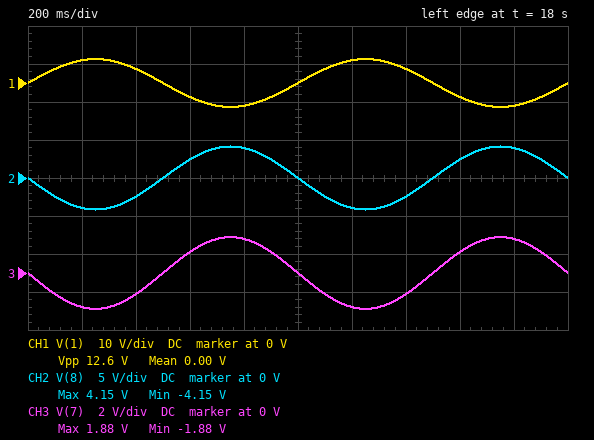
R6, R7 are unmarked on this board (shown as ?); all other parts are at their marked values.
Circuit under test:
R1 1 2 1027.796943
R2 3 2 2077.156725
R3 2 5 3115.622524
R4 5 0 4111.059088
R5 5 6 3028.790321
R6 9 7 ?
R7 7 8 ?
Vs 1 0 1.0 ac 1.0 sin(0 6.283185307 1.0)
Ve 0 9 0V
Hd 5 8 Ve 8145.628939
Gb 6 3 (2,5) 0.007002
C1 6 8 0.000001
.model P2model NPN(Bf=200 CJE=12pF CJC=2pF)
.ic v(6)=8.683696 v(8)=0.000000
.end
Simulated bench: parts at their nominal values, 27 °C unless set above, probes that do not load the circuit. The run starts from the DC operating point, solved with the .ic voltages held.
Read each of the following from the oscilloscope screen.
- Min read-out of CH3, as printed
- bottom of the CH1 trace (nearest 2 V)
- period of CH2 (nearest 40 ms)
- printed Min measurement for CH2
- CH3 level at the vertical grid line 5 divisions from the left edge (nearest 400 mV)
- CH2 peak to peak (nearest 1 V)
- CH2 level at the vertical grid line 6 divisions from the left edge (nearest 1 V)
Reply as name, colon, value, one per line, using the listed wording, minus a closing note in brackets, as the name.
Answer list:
Min read-out of CH3, as printed: -1.88 V
bottom of the CH1 trace: -6 V
period of CH2: 1.00 s
printed Min measurement for CH2: -4.15 V
CH3 level at the vertical grid line 5 divisions from the left edge: 0 V
CH2 peak to peak: 8 V
CH2 level at the vertical grid line 6 divisions from the left edge: -4 V
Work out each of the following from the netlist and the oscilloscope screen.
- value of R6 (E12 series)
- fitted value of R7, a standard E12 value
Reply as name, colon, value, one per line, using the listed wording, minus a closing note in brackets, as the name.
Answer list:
value of R6: 1.5 kΩ
fitted value of R7, a standard E12 value: 1.8 kΩ
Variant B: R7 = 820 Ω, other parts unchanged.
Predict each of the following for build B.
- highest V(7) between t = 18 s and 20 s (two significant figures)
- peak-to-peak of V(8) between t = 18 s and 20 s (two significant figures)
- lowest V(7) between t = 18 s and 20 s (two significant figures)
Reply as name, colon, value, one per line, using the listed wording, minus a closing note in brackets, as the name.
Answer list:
highest V(7) between t = 18 s and 20 s: 1.5 V
peak-to-peak of V(8) between t = 18 s and 20 s: 4.7 V
lowest V(7) between t = 18 s and 20 s: -1.5 V
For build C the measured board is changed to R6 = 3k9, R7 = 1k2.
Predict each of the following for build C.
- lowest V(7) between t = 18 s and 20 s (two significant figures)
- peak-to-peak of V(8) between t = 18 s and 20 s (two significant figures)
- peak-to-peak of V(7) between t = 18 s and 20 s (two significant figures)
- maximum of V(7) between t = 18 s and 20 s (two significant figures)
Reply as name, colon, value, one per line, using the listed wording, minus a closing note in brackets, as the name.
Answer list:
lowest V(7) between t = 18 s and 20 s: -8.7 V
peak-to-peak of V(8) between t = 18 s and 20 s: 23 V
peak-to-peak of V(7) between t = 18 s and 20 s: 17 V
maximum of V(7) between t = 18 s and 20 s: 8.7 V
